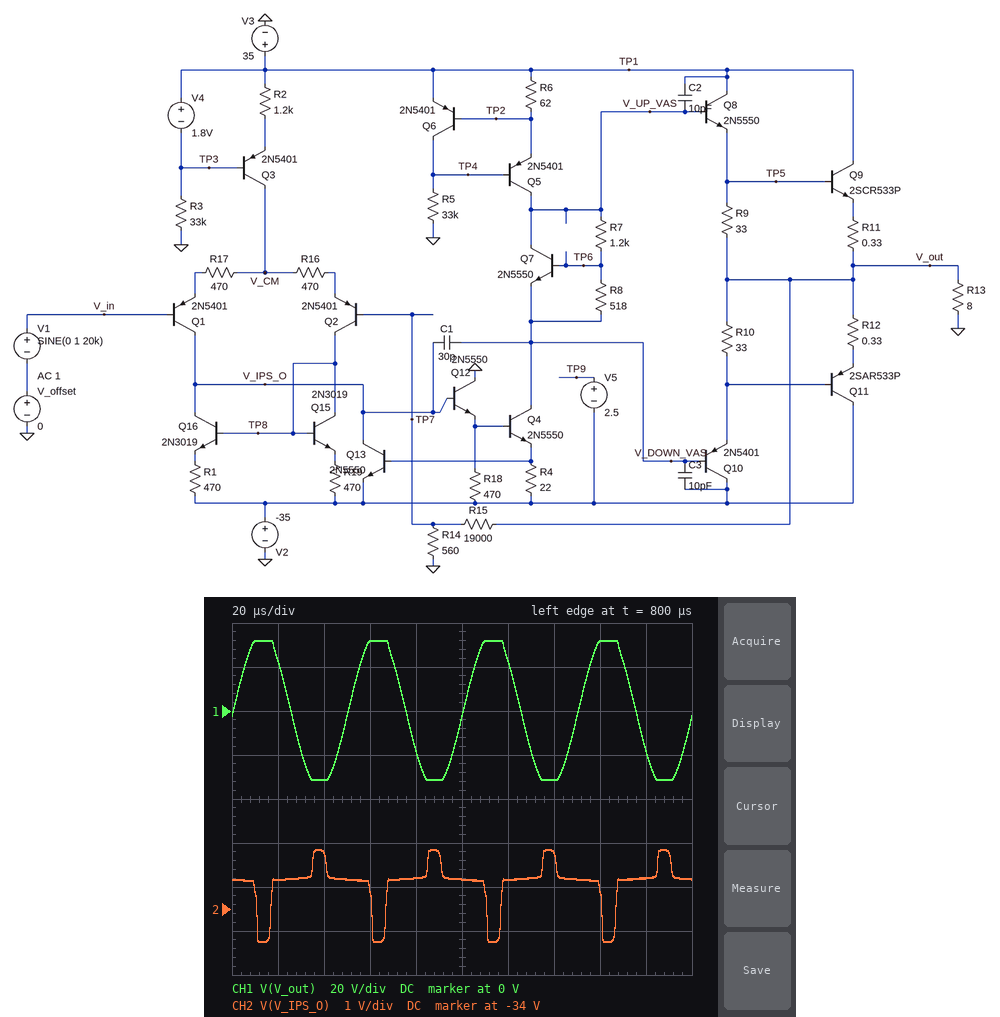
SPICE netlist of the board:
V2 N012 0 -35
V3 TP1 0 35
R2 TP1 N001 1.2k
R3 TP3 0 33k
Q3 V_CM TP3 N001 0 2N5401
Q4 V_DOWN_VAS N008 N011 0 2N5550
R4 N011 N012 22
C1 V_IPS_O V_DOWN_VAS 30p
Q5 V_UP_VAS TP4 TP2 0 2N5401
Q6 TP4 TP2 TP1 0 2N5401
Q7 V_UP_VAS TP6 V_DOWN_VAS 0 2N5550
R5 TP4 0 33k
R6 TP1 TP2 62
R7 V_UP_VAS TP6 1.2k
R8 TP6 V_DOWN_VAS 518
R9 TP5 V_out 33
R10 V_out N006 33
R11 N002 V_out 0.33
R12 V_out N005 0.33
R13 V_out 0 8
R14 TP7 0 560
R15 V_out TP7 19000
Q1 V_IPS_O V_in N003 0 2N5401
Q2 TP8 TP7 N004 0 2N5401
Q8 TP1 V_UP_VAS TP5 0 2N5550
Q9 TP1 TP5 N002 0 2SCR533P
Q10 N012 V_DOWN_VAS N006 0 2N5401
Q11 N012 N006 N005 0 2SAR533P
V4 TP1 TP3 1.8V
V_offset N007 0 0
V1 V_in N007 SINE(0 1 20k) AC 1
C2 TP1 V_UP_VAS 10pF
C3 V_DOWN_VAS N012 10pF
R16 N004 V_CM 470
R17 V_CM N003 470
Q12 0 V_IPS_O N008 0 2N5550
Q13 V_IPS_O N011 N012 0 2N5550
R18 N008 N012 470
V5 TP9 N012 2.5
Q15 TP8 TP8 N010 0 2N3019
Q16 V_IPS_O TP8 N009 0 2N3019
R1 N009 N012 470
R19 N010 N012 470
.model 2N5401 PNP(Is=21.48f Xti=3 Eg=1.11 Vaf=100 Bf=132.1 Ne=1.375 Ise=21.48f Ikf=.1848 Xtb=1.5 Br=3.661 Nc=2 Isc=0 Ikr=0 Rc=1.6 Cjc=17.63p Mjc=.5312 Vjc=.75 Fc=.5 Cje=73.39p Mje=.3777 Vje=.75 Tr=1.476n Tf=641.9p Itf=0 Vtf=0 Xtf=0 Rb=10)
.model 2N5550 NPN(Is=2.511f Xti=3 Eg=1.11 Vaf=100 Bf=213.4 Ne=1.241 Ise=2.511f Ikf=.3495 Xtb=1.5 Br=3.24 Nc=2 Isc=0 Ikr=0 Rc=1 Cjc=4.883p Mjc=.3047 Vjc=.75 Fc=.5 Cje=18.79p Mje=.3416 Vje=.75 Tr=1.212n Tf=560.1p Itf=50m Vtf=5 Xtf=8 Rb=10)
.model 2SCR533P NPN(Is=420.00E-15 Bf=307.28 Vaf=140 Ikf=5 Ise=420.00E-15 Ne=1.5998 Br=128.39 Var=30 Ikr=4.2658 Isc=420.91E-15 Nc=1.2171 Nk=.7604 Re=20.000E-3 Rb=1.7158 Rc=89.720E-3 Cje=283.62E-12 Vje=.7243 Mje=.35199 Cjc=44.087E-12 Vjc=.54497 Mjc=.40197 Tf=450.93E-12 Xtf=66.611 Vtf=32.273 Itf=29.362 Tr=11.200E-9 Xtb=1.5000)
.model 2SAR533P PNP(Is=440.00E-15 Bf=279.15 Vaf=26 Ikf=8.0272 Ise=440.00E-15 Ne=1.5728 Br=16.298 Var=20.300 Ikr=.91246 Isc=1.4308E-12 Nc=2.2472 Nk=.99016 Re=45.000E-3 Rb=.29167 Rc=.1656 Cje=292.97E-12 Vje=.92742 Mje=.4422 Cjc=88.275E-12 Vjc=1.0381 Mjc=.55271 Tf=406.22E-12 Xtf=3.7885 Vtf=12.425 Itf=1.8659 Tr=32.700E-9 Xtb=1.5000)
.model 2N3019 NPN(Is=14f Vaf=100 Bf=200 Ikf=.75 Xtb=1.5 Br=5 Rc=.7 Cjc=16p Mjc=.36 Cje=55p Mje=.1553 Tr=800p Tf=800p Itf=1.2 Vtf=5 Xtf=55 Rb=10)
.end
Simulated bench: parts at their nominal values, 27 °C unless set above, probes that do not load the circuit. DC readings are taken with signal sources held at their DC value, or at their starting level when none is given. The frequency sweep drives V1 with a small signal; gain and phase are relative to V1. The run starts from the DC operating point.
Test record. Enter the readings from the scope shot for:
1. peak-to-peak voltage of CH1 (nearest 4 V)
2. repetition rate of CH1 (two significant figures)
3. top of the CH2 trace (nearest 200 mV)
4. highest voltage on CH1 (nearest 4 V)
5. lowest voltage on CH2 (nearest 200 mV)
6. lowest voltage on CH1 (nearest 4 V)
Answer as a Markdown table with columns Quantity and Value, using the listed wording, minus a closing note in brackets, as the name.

| Quantity | Value |
|---|---|
| peak-to-peak voltage of CH1 | 64 V |
| repetition rate of CH1 | 20 kHz |
| top of the CH2 trace | -32.6 V |
| highest voltage on CH1 | 32 V |
| lowest voltage on CH2 | -34.8 V |
| lowest voltage on CH1 | -32 V |
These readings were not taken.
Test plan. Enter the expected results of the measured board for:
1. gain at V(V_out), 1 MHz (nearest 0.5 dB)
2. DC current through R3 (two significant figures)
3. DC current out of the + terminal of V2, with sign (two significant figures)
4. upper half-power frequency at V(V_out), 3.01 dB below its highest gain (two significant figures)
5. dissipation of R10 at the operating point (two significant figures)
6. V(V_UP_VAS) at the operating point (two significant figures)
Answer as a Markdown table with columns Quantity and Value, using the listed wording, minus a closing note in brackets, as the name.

| Quantity | Value |
|---|---|
| gain at V(V_out), 1 MHz | 18.0 dB |
| DC current through R3 | 1.0 mA |
| DC current out of the + terminal of V2, with sign | -28 mA |
| upper half-power frequency at V(V_out), 3.01 dB below its highest gain | 240 kHz |
| dissipation of R10 at the operating point | 6.9 mW |
| V(V_UP_VAS) at the operating point | 1.5 V |
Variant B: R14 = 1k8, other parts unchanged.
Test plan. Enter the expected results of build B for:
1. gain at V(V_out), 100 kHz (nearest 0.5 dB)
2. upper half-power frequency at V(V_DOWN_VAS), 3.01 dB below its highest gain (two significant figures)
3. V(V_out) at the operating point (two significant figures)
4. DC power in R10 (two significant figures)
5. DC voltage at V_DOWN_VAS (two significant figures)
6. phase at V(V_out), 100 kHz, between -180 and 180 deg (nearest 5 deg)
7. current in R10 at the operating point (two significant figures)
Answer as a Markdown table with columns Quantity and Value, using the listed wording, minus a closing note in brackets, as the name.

| Quantity | Value |
|---|---|
| gain at V(V_out), 100 kHz | 21.0 dB |
| upper half-power frequency at V(V_DOWN_VAS), 3.01 dB below its highest gain | 530 kHz |
| V(V_out) at the operating point | 8.7 mV |
| DC power in R10 | 8.8 mW |
| DC voltage at V_DOWN_VAS | -1.2 V |
| phase at V(V_out), 100 kHz, between -180 and 180 deg | -10 deg |
| current in R10 at the operating point | 16 mA |
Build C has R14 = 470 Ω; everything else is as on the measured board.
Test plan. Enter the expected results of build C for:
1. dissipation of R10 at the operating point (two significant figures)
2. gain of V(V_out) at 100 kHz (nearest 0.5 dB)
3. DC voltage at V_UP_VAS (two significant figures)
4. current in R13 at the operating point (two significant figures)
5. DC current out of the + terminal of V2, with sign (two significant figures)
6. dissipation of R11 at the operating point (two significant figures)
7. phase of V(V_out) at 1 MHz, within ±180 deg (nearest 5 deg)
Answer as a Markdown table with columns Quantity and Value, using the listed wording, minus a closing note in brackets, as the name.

| Quantity | Value |
|---|---|
| dissipation of R10 at the operating point | 6.6 mW |
| gain of V(V_out) at 100 kHz | 31.5 dB |
| DC voltage at V_UP_VAS | 1.6 V |
| current in R13 at the operating point | 24 mA |
| DC current out of the + terminal of V2, with sign | -27 mA |
| dissipation of R11 at the operating point | 120 µW |
| phase of V(V_out) at 1 MHz, within ±180 deg | -90 deg |
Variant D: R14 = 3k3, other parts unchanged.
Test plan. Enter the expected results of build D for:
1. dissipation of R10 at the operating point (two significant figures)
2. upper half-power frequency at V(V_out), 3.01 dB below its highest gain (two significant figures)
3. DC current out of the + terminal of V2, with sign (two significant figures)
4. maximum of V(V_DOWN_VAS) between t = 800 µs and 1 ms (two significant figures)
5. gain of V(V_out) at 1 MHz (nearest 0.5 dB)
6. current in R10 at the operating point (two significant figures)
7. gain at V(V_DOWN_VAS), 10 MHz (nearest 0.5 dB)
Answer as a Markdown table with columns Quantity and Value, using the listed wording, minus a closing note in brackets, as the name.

| Quantity | Value |
|---|---|
| dissipation of R10 at the operating point | 9.6 mW |
| upper half-power frequency at V(V_out), 3.01 dB below its highest gain | 1.1 MHz |
| DC current out of the + terminal of V2, with sign | -33 mA |
| maximum of V(V_DOWN_VAS) between t = 800 µs and 1 ms | 6.0 V |
| gain of V(V_out) at 1 MHz | 14.0 dB |
| current in R10 at the operating point | 17 mA |
| gain at V(V_DOWN_VAS), 10 MHz | -8.5 dB |
